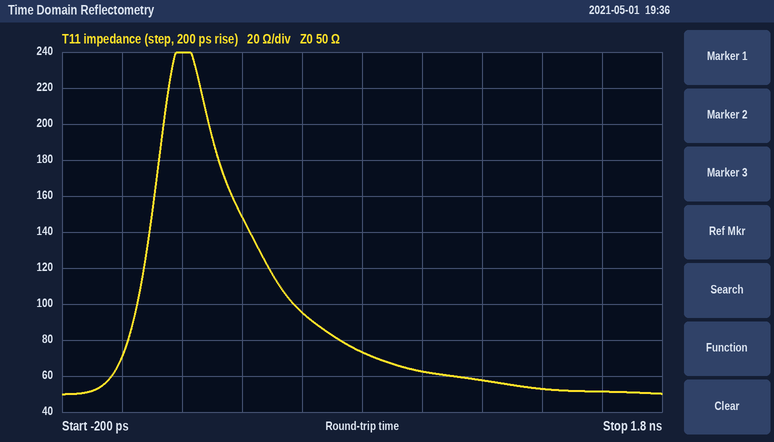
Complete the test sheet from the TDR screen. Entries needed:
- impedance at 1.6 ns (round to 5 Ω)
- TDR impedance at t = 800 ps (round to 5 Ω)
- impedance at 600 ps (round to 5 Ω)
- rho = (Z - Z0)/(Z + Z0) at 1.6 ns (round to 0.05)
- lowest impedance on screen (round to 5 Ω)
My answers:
50 Ω
75 Ω
95 Ω
0.00
50 Ω
